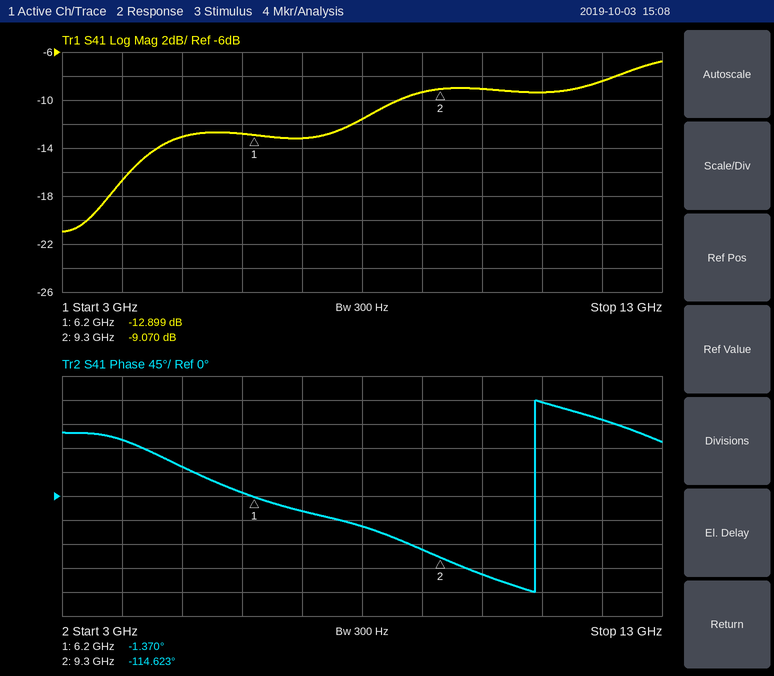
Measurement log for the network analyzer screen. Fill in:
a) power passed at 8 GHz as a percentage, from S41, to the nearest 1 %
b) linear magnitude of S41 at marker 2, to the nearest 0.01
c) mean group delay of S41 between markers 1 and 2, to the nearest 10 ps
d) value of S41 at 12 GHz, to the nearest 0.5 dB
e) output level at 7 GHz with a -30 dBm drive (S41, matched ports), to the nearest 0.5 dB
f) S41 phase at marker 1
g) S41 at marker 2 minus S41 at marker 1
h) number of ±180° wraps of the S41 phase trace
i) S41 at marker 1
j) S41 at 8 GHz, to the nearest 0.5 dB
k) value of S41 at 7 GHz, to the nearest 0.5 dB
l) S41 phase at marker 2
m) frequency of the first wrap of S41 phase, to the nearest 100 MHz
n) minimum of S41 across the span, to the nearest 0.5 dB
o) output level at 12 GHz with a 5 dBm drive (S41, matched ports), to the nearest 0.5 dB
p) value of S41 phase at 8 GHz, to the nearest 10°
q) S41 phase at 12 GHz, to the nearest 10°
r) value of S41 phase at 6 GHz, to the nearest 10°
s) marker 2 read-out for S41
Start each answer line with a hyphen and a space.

- 7 %
- 0.35
- 100 ps
- -8.5 dB
- -43.0 dBm
- -1.370°
- 3.829 dB
- 1
- -12.899 dB
- -11.5 dB
- -13.0 dB
- -114.623°
- 10.9 GHz
- -21.0 dB
- -3.5 dBm
- -60°
- 140°
- 10°
- -9.070 dB
